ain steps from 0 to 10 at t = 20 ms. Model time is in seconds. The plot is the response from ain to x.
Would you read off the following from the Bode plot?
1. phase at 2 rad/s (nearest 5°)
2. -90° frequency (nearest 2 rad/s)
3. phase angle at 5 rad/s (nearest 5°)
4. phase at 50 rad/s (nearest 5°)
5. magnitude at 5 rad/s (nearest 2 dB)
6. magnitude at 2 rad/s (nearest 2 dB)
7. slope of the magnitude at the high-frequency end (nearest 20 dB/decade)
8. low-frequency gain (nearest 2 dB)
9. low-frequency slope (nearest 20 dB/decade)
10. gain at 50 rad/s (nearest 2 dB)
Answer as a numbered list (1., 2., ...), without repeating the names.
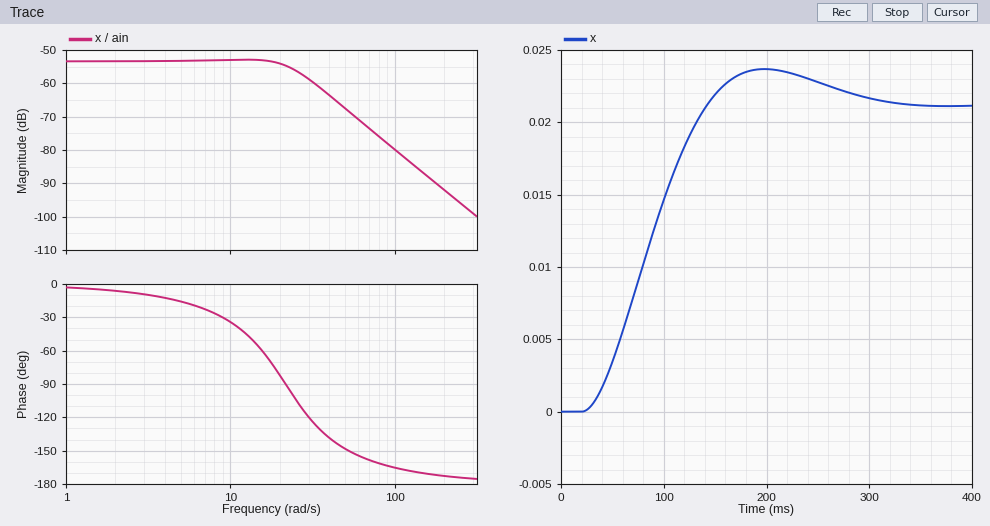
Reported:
1. -5°
2. 22 rad/s
3. -15°
4. -150°
5. -54 dB
6. -54 dB
7. -40 dB/decade
8. -54 dB
9. 0 dB/decade
10. -68 dB
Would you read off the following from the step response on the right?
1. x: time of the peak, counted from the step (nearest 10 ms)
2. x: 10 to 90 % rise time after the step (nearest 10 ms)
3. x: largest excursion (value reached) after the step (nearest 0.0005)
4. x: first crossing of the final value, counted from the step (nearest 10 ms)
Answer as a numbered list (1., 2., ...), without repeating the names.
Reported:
1. 180 ms
2. 80 ms
3. 0.0235
4. 120 ms
